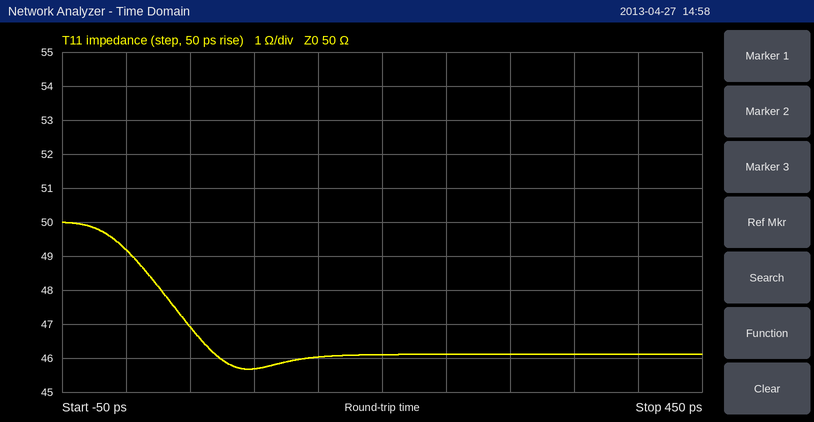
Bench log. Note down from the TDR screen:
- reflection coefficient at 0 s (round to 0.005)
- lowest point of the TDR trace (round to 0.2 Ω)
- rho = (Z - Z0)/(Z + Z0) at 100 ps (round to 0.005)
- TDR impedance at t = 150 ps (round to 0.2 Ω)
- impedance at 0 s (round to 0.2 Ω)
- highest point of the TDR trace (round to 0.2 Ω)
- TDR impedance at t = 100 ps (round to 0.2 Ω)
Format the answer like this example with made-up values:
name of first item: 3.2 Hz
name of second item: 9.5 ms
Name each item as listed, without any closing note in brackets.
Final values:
reflection coefficient at 0 s: -0.010
lowest point of the TDR trace: 45.6 Ω
rho = (Z - Z0)/(Z + Z0) at 100 ps: -0.045
TDR impedance at t = 150 ps: 46.0 Ω
impedance at 0 s: 49.2 Ω
highest point of the TDR trace: 50.0 Ω
TDR impedance at t = 100 ps: 45.6 Ω
